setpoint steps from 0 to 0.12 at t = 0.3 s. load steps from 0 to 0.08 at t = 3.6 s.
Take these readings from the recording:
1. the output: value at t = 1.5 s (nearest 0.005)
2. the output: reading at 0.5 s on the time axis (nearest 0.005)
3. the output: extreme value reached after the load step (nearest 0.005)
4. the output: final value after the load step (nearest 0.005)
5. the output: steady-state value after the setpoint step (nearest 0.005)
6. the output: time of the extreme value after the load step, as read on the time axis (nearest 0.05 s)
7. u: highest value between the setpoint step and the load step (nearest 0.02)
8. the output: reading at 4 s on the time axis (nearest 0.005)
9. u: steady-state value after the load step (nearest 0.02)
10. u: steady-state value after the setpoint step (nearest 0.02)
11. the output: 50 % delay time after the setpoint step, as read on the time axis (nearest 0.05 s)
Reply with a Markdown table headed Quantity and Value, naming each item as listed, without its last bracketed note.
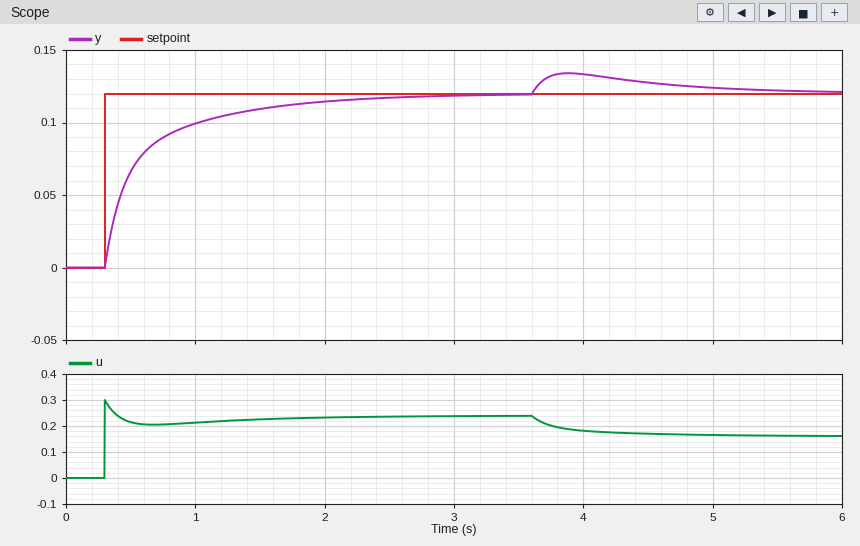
| Quantity | Value |
|---|---|
| the output: value at t = 1.5 s | 0.110 |
| the output: reading at 0.5 s on the time axis | 0.065 |
| the output: extreme value reached after the load step | 0.135 |
| the output: final value after the load step | 0.120 |
| the output: steady-state value after the setpoint step | 0.120 |
| the output: time of the extreme value after the load step, as read on the time axis | 3.90 s |
| u: highest value between the setpoint step and the load step | 0.30 |
| the output: reading at 4 s on the time axis | 0.135 |
| u: steady-state value after the load step | 0.16 |
| u: steady-state value after the setpoint step | 0.24 |
| the output: 50 % delay time after the setpoint step, as read on the time axis | 0.45 s |
